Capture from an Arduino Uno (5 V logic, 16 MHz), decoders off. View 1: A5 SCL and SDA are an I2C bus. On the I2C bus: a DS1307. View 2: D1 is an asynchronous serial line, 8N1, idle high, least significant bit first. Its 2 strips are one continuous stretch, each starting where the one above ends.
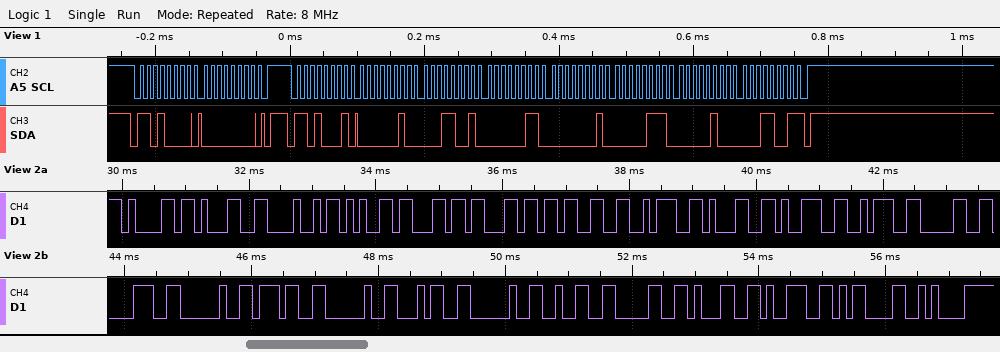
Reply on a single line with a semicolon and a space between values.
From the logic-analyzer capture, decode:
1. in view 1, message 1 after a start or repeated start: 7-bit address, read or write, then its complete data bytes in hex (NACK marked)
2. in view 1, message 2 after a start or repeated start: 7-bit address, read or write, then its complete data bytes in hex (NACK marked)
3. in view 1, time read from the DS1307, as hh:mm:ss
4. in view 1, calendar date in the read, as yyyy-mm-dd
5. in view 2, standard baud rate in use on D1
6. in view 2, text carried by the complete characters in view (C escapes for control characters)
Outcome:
0x68 write: 00; 0x68 read: 02 19 03 01 07 04 19 NACK; 03:19:02; 2019-04-07; 9600 baud; "a1Hell3:19:08 7 4 2019\r\n"
